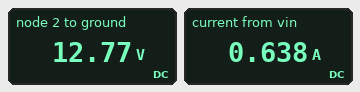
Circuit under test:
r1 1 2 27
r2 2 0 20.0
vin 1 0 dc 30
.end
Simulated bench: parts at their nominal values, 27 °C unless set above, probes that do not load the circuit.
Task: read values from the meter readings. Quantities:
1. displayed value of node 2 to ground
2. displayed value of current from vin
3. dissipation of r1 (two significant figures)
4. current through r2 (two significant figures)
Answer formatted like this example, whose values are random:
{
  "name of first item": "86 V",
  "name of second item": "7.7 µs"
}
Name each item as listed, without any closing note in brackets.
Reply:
{
  "displayed value of node 2 to ground": "12.77 V",
  "displayed value of current from vin": "0.638 A",
  "dissipation of r1": "11 W",
  "current through r2": "640 mA"
}
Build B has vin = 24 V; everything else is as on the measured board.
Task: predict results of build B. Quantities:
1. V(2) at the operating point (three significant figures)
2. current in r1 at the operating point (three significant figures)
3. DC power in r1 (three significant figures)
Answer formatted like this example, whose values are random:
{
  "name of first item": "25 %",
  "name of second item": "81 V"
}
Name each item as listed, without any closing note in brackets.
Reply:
{
  "V(2) at the operating point": "10.2 V",
  "current in r1 at the operating point": "511 mA",
  "DC power in r1": "7.04 W"
}
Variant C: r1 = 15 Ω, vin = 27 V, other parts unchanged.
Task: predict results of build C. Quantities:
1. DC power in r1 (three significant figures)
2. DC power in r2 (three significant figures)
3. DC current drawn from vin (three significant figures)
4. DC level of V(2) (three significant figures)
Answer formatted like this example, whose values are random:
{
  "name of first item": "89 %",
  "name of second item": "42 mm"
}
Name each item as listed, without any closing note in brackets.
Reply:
{
  "DC power in r1": "8.93 W",
  "DC power in r2": "11.9 W",
  "DC current drawn from vin": "771 mA",
  "DC level of V(2)": "15.4 V"
}
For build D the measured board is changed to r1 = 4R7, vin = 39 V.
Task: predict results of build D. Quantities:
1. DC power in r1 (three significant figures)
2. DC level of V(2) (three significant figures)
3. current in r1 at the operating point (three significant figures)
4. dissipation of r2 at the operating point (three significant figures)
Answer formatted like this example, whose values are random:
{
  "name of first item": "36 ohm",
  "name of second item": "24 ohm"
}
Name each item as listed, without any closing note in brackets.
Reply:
{
  "DC power in r1": "11.7 W",
  "DC level of V(2)": "31.6 V",
  "current in r1 at the operating point": "1.58 A",
  "dissipation of r2 at the operating point": "49.9 W"
}
